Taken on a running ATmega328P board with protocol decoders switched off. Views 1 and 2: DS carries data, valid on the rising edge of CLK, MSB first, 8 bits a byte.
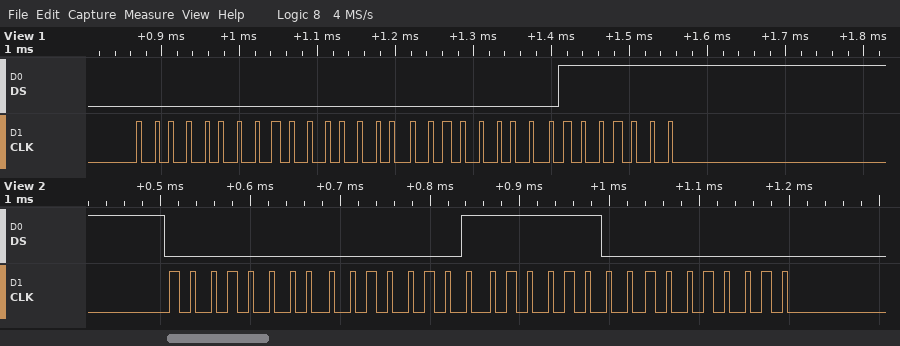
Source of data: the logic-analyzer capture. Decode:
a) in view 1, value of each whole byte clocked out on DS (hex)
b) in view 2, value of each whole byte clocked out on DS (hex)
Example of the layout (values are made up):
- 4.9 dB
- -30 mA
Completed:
- 00 00 00 7F
- 0x00 0x01 0xFC 0x00
